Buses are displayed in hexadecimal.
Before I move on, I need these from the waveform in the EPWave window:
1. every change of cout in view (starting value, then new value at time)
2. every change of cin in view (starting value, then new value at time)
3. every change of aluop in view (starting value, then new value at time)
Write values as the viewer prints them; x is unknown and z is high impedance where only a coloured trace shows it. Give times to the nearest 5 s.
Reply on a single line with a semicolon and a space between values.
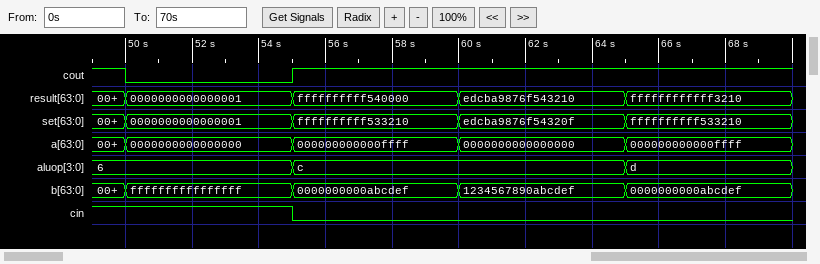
1, 0 at 50 s, 1 at 55 s; 1, 0 at 55 s; 6, c at 55 s, d at 65 s
